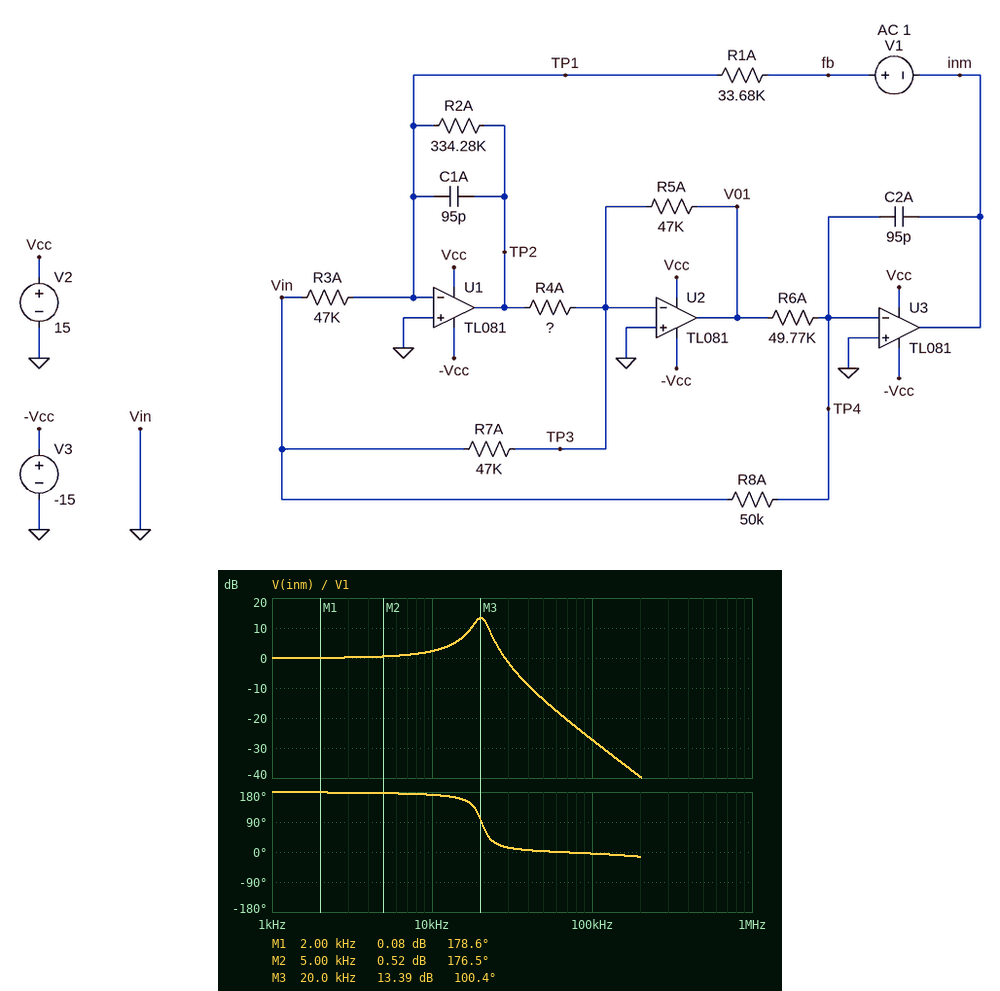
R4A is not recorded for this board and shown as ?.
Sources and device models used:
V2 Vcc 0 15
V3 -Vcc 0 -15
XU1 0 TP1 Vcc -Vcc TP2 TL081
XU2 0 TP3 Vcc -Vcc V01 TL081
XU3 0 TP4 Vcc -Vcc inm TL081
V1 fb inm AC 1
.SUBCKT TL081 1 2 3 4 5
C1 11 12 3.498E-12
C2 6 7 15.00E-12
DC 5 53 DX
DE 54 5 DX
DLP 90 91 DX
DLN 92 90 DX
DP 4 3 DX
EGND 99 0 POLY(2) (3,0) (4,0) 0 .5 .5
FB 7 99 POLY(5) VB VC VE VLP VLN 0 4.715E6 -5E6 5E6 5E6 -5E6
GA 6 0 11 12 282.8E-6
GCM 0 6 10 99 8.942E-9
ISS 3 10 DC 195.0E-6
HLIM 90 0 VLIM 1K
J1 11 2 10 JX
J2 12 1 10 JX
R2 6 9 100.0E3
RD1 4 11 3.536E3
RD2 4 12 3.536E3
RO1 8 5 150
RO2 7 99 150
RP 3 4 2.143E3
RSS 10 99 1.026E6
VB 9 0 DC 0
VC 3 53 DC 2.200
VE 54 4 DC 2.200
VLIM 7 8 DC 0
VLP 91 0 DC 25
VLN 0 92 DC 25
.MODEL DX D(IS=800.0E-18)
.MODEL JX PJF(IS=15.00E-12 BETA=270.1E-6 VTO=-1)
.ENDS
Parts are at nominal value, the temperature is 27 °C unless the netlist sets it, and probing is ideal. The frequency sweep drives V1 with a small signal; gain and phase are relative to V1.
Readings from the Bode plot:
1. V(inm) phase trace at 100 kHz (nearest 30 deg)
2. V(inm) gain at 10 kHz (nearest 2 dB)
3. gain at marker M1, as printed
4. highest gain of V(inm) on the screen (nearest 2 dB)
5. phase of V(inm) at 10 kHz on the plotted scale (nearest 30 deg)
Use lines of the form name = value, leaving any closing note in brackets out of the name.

V(inm) phase trace at 100 kHz = 0 deg
V(inm) gain at 10 kHz = 2 dB
gain at marker M1, as printed = 0.08 dB
highest gain of V(inm) on the screen = 14 dB
phase of V(inm) at 10 kHz on the plotted scale = 180 deg
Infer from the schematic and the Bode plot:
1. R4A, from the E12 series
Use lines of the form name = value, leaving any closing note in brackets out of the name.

R4A, from the E12 series = 180 kΩ
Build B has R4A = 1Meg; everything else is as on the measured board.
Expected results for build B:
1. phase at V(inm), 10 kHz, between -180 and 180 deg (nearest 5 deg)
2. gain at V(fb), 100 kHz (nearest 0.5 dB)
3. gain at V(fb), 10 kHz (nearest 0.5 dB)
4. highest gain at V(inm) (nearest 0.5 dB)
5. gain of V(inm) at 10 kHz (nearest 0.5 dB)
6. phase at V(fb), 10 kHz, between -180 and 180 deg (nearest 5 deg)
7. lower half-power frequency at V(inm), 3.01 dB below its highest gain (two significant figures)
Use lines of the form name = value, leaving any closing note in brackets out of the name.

phase at V(inm), 10 kHz, between -180 and 180 deg = 60 deg
gain at V(fb), 100 kHz = 0 dB
gain at V(fb), 10 kHz = 6.5 dB
highest gain at V(inm) = 5.5 dB
gain of V(inm) at 10 kHz = 3.0 dB
phase at V(fb), 10 kHz, between -180 and 180 deg = 35 deg
lower half-power frequency at V(inm), 3.01 dB below its highest gain = 4.9 kHz
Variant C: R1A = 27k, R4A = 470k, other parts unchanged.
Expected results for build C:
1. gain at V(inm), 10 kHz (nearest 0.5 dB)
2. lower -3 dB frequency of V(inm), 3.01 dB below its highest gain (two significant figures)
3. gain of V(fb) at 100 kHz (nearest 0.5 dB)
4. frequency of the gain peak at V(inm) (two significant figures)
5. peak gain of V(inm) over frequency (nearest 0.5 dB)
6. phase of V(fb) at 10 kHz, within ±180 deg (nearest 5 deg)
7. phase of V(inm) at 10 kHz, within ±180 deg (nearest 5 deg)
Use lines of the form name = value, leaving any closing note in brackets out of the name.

gain at V(inm), 10 kHz = 5.0 dB
lower -3 dB frequency of V(inm), 3.01 dB below its highest gain = 11 kHz
gain of V(fb) at 100 kHz = 0 dB
frequency of the gain peak at V(inm) = 14 kHz
peak gain of V(inm) over frequency = 10.0 dB
phase of V(fb) at 10 kHz, within ±180 deg = 130 deg
phase of V(inm) at 10 kHz, within ±180 deg = 155 deg
